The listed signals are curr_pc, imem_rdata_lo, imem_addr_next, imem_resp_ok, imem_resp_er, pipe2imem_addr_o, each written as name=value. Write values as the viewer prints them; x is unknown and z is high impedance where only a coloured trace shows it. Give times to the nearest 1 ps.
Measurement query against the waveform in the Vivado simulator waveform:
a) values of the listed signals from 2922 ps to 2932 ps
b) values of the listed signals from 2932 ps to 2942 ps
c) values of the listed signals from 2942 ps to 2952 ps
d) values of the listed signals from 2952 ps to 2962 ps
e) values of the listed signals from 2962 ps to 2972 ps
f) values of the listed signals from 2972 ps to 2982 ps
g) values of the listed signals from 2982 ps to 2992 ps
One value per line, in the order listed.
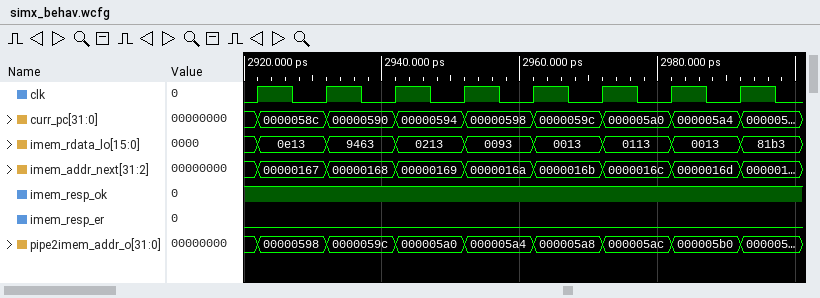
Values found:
curr_pc=0000058c, imem_rdata_lo=0e13, imem_addr_next=00000167, imem_resp_ok=1, imem_resp_er=0, pipe2imem_addr_o=00000598
curr_pc=00000590, imem_rdata_lo=9463, imem_addr_next=00000168, imem_resp_ok=1, imem_resp_er=0, pipe2imem_addr_o=0000059c
curr_pc=00000594, imem_rdata_lo=0213, imem_addr_next=00000169, imem_resp_ok=1, imem_resp_er=0, pipe2imem_addr_o=000005a0
curr_pc=00000598, imem_rdata_lo=0093, imem_addr_next=0000016a, imem_resp_ok=1, imem_resp_er=0, pipe2imem_addr_o=000005a4
curr_pc=0000059c, imem_rdata_lo=0013, imem_addr_next=0000016b, imem_resp_ok=1, imem_resp_er=0, pipe2imem_addr_o=000005a8
curr_pc=000005a0, imem_rdata_lo=0113, imem_addr_next=0000016c, imem_resp_ok=1, imem_resp_er=0, pipe2imem_addr_o=000005ac
curr_pc=000005a4, imem_rdata_lo=0013, imem_addr_next=0000016d, imem_resp_ok=1, imem_resp_er=0, pipe2imem_addr_o=000005b0
